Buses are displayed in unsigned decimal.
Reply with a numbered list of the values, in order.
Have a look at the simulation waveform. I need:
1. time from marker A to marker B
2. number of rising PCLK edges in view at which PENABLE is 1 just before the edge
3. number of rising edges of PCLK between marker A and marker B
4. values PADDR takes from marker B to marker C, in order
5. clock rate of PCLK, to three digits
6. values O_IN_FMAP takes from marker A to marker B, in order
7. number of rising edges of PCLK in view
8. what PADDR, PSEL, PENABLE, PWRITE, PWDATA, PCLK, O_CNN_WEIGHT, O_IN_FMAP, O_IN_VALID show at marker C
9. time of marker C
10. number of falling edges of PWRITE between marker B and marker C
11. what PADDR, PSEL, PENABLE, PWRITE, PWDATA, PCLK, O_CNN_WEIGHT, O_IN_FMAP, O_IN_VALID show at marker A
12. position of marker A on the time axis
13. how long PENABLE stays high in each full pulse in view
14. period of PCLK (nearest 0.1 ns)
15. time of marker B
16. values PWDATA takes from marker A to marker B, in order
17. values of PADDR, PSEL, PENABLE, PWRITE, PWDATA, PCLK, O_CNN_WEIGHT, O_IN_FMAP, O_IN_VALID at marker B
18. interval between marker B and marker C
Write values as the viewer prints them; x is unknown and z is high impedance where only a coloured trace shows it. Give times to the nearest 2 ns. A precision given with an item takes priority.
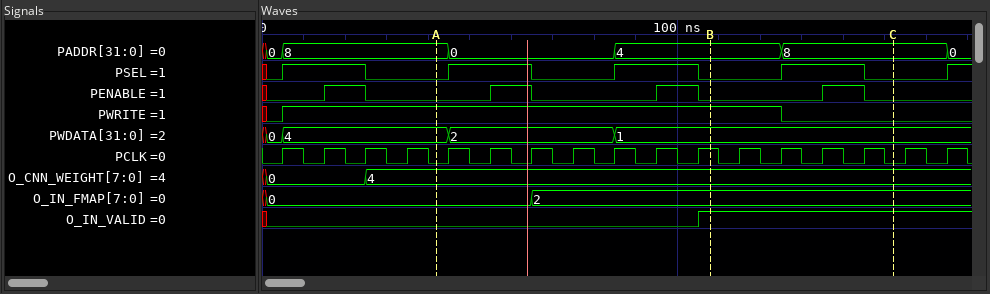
1. 66 ns
2. 4
3. 7
4. 4, 8
5. 100 MHz
6. 0, 2
7. 17
8. PADDR=8, PSEL=0, PENABLE=0, PWRITE=0, PWDATA=1, PCLK=0, O_CNN_WEIGHT=4, O_IN_FMAP=2, O_IN_VALID=1
9. 152 ns
10. 1
11. PADDR=8, PSEL=0, PENABLE=0, PWRITE=1, PWDATA=4, PCLK=0, O_CNN_WEIGHT=4, O_IN_FMAP=0, O_IN_VALID=0
12. 42 ns
13. 10 ns, 10 ns, 10 ns, 10 ns
14. 10 ns
15. 108 ns
16. 4, 2, 1
17. PADDR=4, PSEL=0, PENABLE=0, PWRITE=1, PWDATA=1, PCLK=1, O_CNN_WEIGHT=4, O_IN_FMAP=2, O_IN_VALID=1
18. 44 ns
